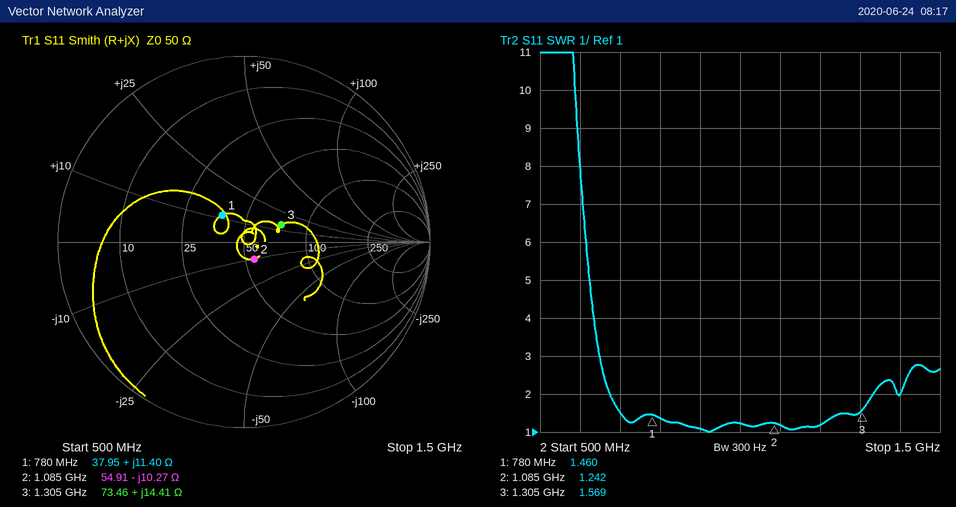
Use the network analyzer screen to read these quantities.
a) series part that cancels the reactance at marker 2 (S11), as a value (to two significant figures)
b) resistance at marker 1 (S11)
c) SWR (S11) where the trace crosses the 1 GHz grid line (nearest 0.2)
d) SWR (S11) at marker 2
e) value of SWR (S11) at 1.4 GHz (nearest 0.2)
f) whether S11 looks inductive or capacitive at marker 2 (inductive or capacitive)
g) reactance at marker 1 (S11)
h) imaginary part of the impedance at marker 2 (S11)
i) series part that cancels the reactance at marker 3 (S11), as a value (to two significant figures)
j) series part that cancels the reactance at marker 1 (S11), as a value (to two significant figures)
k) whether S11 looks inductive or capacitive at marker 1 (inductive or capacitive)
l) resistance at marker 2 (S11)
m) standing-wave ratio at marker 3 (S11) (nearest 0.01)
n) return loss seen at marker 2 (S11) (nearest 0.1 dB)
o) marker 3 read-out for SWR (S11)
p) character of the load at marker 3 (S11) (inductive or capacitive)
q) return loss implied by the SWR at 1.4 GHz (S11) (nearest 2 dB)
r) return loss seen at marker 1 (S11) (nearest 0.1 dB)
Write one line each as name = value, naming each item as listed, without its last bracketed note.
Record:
series part that cancels the reactance at marker 2 (S11), as a value = 1.5 nH
resistance at marker 1 = 37.95 Ω
SWR (S11) where the trace crosses the 1 GHz grid line = 1.2
SWR (S11) at marker 2 = 1.242
value of SWR (S11) at 1.4 GHz = 2.0
whether S11 looks inductive or capacitive at marker 2 = capacitive
reactance at marker 1 = +11.40 Ω
imaginary part of the impedance at marker 2 = -10.27 Ω
series part that cancels the reactance at marker 3 (S11), as a value = 8.5 pF
series part that cancels the reactance at marker 1 (S11), as a value = 18 pF
whether S11 looks inductive or capacitive at marker 1 = inductive
resistance at marker 2 = 54.91 Ω
standing-wave ratio at marker 3 (S11) = 1.57
return loss seen at marker 2 (S11) = 19.3 dB
marker 3 read-out for SWR = 1.569
character of the load at marker 3 (S11) = inductive
return loss implied by the SWR at 1.4 GHz (S11) = 10 dB
return loss seen at marker 1 (S11) = 14.6 dB
